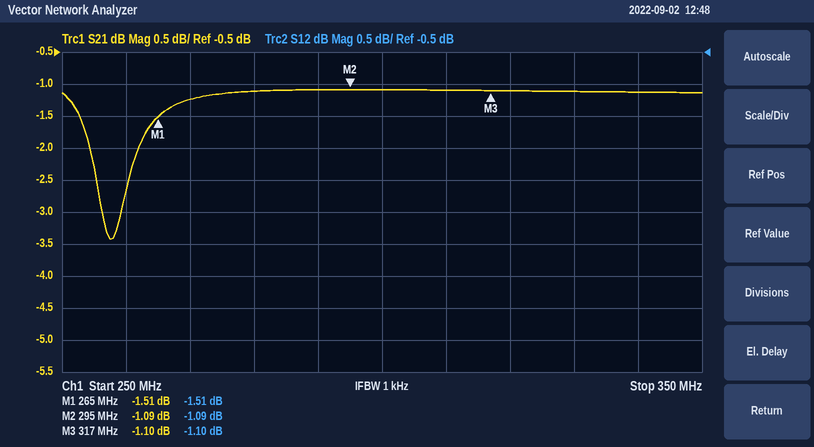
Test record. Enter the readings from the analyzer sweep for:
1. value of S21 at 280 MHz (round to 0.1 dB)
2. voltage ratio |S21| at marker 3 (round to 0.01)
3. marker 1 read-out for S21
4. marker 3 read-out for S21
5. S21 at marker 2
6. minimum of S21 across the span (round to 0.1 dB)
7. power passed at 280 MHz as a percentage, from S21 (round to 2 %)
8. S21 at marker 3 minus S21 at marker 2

-1.1 dB
0.88
-1.51 dB
-1.10 dB
-1.09 dB
-3.4 dB
78 %
-0.01 dB
